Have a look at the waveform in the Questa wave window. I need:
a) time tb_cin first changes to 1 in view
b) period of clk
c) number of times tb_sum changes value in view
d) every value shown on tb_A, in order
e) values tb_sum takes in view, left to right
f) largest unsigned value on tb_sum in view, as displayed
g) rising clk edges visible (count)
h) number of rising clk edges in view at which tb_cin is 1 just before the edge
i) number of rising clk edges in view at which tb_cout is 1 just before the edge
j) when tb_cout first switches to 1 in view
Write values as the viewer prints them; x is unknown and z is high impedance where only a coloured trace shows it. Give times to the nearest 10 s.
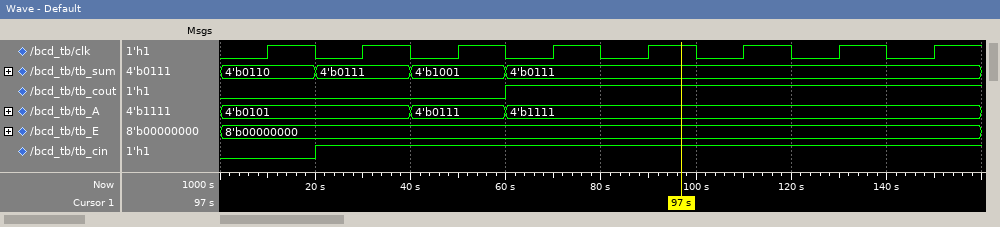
20 s
20 s
3
4'b0101, 4'b0111, 4'b1111
4'b0110, 4'b0111, 4'b1001, 4'b0111
4'b1001
8
7
5
60 s
